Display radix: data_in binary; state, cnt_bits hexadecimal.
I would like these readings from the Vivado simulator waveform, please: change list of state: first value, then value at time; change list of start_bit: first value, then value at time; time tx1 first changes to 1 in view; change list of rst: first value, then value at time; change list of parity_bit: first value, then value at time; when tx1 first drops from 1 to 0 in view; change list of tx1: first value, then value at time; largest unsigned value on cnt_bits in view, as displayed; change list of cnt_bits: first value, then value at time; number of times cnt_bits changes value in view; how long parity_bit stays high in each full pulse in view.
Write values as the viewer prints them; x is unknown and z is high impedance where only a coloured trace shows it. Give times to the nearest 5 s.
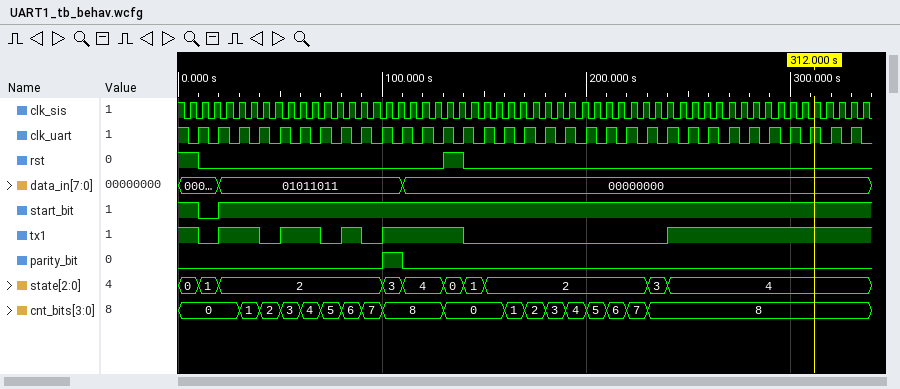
0, 1 at 10 s, 2 at 20 s, 3 at 100 s, 4 at 110 s, 0 at 130 s, 1 at 140 s, 2 at 150 s, 3 at 230 s, 4 at 240 s
1, 0 at 10 s, 1 at 20 s
20 s
1, 0 at 10 s, 1 at 130 s, 0 at 140 s
0, 1 at 100 s, 0 at 110 s
10 s
1, 0 at 10 s, 1 at 20 s, 0 at 40 s, 1 at 50 s, 0 at 70 s, 1 at 80 s, 0 at 90 s, 1 at 100 s, 0 at 140 s, 1 at 240 s
8
0, 1 at 30 s, 2 at 40 s, 3 at 50 s, 4 at 60 s, 5 at 70 s, 6 at 80 s, 7 at 90 s, 8 at 100 s, 0 at 130 s, 1 at 160 s, 2 at 170 s, 3 at 180 s, 4 at 190 s, 5 at 200 s, 6 at 210 s, 7 at 220 s, 8 at 230 s
17
10 s
